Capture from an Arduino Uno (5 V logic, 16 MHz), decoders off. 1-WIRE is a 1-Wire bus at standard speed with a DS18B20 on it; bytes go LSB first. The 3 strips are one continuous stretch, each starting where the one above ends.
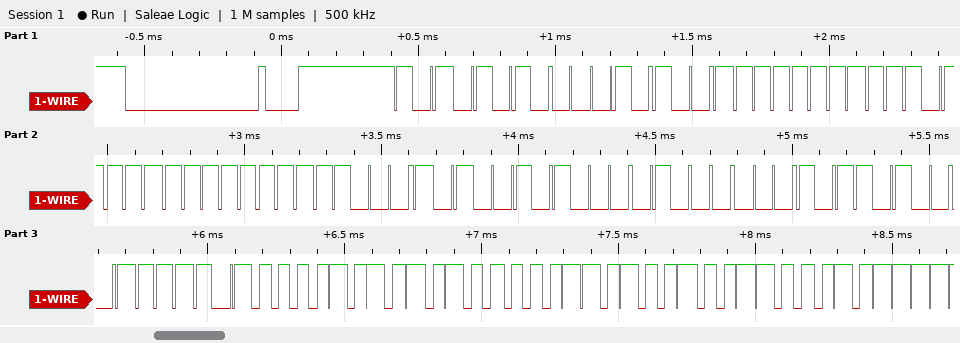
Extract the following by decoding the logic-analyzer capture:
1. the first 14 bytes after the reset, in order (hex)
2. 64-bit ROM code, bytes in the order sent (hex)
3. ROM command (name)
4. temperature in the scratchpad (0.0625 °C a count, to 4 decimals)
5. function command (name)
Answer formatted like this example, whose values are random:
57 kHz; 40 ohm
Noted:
55 28 FF F7 FF A3 14 02 2D BE 50 05 4B 46; 28 FF F7 FF A3 14 02 2D; Match ROM; 85.0000 °C; Read Scratchpad
